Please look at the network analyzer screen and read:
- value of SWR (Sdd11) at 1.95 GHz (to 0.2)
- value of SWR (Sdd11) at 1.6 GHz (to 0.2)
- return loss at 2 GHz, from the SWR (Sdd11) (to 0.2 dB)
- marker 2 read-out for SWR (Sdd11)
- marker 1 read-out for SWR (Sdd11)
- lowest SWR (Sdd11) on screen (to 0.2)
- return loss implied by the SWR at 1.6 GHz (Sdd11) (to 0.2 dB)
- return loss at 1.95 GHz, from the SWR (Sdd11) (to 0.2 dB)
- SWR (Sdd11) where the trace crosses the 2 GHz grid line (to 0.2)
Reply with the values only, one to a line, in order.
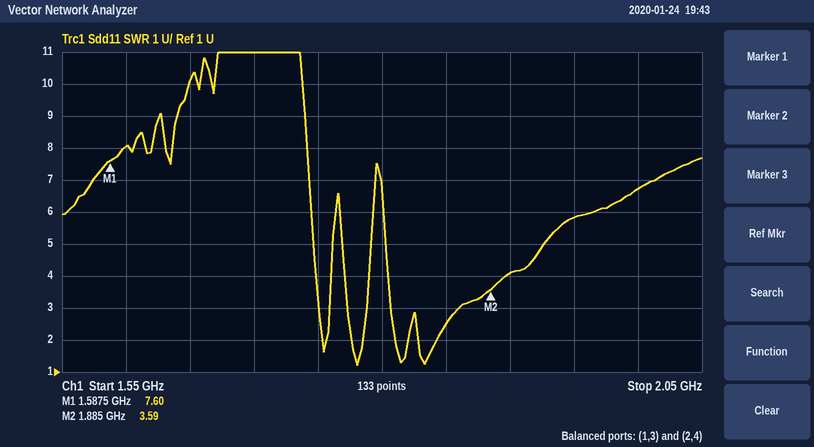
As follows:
5.8
8.0
2.6 dB
3.59
7.60
1.2
2.2 dB
3.0 dB
6.8
